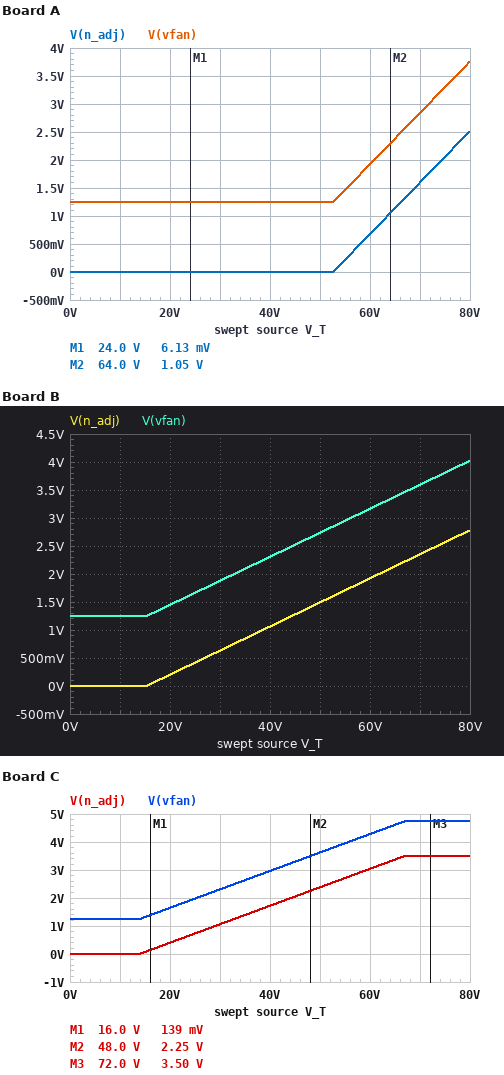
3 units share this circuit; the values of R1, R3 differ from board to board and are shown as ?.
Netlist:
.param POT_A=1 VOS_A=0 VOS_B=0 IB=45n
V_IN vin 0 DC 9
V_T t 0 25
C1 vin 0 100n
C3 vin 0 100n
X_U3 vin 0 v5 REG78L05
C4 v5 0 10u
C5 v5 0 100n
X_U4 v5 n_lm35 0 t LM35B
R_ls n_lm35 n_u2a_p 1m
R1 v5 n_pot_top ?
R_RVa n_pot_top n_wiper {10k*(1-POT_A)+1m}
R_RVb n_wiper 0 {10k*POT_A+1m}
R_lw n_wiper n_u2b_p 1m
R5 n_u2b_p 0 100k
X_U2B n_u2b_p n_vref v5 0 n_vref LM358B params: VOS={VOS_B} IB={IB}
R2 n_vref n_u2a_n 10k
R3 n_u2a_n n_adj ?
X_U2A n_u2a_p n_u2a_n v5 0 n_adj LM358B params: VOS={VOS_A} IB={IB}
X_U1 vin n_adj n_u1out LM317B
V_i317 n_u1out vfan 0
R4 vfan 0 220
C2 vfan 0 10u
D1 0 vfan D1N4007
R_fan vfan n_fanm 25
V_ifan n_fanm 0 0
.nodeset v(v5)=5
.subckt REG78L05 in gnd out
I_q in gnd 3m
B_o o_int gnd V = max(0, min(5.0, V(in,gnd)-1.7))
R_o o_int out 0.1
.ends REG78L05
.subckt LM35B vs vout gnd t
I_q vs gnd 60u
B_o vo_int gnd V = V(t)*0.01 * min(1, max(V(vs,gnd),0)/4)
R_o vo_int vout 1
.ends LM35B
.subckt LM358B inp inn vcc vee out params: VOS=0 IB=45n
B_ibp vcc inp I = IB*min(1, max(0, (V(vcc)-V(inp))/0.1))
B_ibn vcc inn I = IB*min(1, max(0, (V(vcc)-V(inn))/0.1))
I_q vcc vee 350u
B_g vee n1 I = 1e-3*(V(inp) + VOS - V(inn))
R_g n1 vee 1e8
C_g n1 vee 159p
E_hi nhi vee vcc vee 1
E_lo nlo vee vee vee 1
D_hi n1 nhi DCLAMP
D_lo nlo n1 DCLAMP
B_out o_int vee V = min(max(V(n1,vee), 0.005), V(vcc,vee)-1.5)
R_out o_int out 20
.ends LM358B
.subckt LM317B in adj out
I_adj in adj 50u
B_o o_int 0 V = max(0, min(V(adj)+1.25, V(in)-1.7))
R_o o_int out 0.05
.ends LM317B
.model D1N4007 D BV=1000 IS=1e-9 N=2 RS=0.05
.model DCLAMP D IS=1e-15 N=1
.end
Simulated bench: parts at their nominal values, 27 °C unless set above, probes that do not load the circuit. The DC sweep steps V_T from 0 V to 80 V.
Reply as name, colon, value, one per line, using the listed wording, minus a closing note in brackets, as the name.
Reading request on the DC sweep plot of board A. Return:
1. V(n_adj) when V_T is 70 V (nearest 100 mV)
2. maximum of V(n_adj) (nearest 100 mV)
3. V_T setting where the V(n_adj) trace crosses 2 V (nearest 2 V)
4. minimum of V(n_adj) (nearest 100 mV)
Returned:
V(n_adj) when V_T is 70 V: 1.6 V
maximum of V(n_adj): 2.5 V
V_T setting where the V(n_adj) trace crosses 2 V: 74 V
minimum of V(n_adj): 0 V
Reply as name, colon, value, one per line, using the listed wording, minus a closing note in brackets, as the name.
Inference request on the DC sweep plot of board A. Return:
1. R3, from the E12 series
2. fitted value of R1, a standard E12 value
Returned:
R3, from the E12 series: 82 kΩ
fitted value of R1, a standard E12 value: 68 kΩ
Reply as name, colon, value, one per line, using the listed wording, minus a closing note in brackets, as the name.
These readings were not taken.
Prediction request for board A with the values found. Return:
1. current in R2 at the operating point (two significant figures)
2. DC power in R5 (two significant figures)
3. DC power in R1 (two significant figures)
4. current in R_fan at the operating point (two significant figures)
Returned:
current in R2 at the operating point: 6.3 µA
DC power in R5: 3.5 µW
DC power in R1: 290 µW
current in R_fan at the operating point: 50 mA
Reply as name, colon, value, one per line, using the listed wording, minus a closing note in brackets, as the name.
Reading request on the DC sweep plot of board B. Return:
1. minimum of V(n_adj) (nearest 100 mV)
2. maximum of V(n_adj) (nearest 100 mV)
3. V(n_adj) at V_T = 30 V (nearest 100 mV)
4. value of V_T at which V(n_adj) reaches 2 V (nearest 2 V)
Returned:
minimum of V(n_adj): 0 V
maximum of V(n_adj): 2.8 V
V(n_adj) at V_T = 30 V: 600 mV
value of V_T at which V(n_adj) reaches 2 V: 62 V
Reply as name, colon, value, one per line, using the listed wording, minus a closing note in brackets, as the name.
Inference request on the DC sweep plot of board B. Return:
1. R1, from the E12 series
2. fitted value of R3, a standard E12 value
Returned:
R1, from the E12 series: 220 kΩ
fitted value of R3, a standard E12 value: 33 kΩ
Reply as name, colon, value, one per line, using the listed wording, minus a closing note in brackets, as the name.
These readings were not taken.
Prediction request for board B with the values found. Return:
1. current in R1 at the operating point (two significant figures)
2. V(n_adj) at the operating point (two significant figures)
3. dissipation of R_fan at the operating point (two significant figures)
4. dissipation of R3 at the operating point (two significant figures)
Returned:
current in R1 at the operating point: 22 µA
V(n_adj) at the operating point: 420 mV
dissipation of R_fan at the operating point: 110 mW
dissipation of R3 at the operating point: 850 nW
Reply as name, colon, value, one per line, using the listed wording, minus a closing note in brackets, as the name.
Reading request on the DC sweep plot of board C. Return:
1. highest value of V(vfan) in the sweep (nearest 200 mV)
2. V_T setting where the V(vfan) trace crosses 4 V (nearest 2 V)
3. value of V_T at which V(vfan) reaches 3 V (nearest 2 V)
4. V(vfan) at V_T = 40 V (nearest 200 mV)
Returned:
highest value of V(vfan) in the sweep: 4.8 V
V_T setting where the V(vfan) trace crosses 4 V: 56 V
value of V_T at which V(vfan) reaches 3 V: 40 V
V(vfan) at V_T = 40 V: 3.0 V
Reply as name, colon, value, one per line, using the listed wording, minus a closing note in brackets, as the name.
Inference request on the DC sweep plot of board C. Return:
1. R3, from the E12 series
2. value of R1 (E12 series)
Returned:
R3, from the E12 series: 56 kΩ
value of R1: 270 kΩ
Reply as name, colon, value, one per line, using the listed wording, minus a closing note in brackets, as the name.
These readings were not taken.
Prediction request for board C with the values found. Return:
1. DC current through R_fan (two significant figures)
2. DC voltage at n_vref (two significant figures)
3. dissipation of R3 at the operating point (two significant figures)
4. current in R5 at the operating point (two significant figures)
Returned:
DC current through R_fan: 79 mA
DC voltage at n_vref: 160 mV
dissipation of R3 at the operating point: 4.2 µW
current in R5 at the operating point: 1.6 µA
